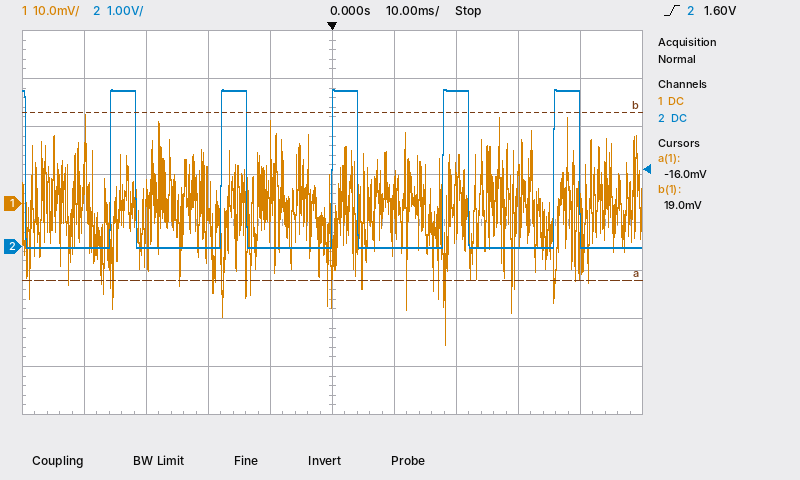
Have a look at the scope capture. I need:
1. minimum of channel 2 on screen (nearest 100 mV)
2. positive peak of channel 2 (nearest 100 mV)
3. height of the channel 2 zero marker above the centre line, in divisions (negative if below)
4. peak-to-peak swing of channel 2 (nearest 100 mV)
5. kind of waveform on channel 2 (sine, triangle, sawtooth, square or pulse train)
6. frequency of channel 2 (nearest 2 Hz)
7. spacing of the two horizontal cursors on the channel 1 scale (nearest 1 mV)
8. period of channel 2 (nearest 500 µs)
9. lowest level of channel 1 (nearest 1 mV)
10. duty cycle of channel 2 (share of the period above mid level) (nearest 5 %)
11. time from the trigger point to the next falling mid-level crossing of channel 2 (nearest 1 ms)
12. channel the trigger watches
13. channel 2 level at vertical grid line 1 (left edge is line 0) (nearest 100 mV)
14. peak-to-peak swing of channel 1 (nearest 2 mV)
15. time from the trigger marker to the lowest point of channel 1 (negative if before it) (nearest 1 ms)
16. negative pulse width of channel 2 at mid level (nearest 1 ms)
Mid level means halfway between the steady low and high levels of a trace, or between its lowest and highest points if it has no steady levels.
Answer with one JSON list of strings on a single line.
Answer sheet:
["0.0 V", "3.3 V", "-0.5 div", "3.3 V", "pulse train", "56 Hz", "35 mV", "18.0 ms", "-29 mV", "25 %", "4 ms", "channel 2", "0.0 V", "48 mV", "+18 ms", "14 ms"]
